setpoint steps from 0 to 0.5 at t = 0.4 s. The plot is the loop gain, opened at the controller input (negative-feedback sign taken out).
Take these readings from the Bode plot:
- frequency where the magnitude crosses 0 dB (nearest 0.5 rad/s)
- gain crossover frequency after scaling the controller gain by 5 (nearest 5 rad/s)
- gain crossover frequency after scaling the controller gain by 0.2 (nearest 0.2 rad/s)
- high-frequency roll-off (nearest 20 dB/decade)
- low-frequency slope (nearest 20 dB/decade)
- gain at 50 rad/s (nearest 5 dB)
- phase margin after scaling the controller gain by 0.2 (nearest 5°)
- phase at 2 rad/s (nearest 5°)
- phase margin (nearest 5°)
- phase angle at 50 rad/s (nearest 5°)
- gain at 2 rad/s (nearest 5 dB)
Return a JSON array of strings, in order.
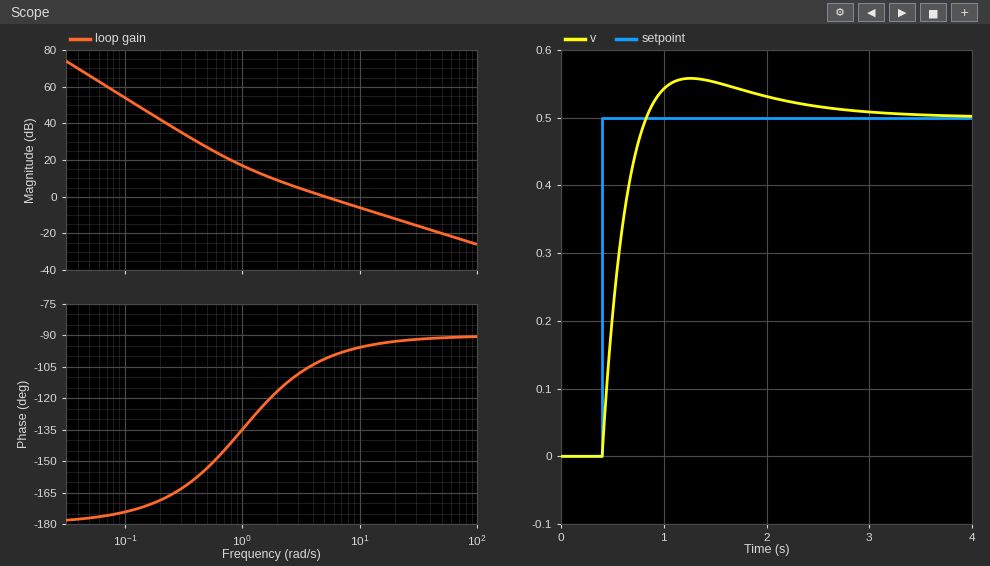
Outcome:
["5.0 rad/s", "25 rad/s", "1.2 rad/s", "-20 dB/decade", "-40 dB/decade", "-20 dB", "50°", "-115°", "80°", "-90°", "10 dB"]
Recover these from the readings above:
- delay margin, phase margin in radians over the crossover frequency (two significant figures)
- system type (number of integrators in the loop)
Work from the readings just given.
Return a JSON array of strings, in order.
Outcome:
["0.28 s", "2"]
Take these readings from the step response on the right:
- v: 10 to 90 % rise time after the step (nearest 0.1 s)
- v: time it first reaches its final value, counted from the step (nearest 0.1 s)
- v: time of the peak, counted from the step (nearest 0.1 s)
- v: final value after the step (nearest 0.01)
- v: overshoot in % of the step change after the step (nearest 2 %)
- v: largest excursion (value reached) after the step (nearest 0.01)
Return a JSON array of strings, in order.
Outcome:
["0.3 s", "0.4 s", "0.9 s", "0.50", "12 %", "0.56"]
